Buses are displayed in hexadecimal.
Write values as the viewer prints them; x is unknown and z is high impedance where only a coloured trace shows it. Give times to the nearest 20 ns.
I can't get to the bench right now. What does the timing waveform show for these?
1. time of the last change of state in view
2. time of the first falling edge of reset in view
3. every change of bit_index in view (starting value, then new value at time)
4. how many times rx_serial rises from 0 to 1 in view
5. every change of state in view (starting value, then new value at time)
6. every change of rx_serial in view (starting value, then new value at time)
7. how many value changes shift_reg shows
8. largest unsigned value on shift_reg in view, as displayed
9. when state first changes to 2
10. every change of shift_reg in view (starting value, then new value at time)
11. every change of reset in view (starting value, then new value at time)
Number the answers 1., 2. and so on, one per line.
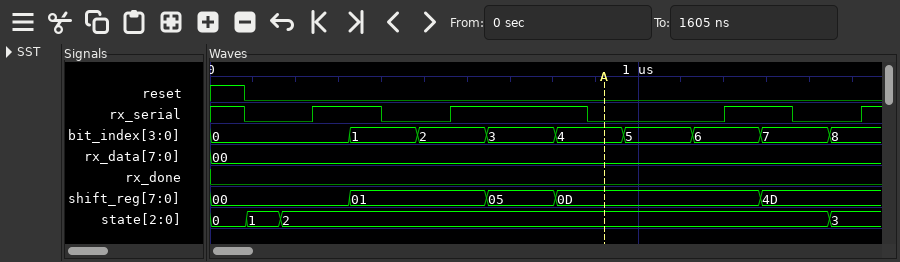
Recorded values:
1. 1440 ns
2. 80 ns
3. 0, 1 at 320 ns, 2 at 480 ns, 3 at 640 ns, 4 at 800 ns, 5 at 960 ns, 6 at 1120 ns, 7 at 1280 ns, 8 at 1440 ns
4. 4
5. 0, 1 at 80 ns, 2 at 160 ns, 3 at 1440 ns
6. 1, 0 at 80 ns, 1 at 240 ns, 0 at 400 ns, 1 at 560 ns, 0 at 880 ns, 1 at 1200 ns, 0 at 1360 ns, 1 at 1520 ns
7. 4
8. 4D
9. 160 ns
10. 00, 01 at 320 ns, 05 at 640 ns, 0D at 800 ns, 4D at 1280 ns
11. 1, 0 at 80 ns
